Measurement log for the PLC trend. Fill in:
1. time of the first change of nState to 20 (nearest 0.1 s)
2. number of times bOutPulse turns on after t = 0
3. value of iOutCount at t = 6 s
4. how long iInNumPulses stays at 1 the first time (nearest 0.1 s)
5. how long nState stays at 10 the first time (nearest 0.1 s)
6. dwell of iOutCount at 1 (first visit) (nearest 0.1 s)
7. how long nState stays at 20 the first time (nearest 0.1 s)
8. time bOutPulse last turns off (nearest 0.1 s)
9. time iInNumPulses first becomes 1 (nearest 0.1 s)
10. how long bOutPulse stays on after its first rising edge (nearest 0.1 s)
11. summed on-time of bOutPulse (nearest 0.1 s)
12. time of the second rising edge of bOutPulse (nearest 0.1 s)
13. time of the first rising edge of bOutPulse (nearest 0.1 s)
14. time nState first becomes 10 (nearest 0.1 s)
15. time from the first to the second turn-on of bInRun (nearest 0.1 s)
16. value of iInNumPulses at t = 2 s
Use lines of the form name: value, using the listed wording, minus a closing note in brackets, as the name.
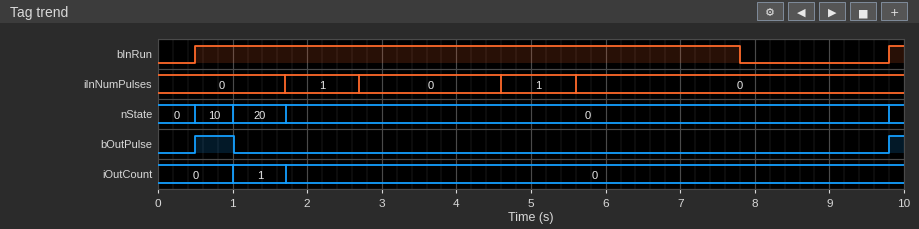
time of the first change of nState to 20: 1.0 s
number of times bOutPulse turns on after t = 0: 2
value of iOutCount at t = 6 s: 0
how long iInNumPulses stays at 1 the first time: 1.0 s
how long nState stays at 10 the first time: 0.5 s
dwell of iOutCount at 1 (first visit): 0.7 s
how long nState stays at 20 the first time: 0.7 s
time bOutPulse last turns off: 1.0 s
time iInNumPulses first becomes 1: 1.7 s
how long bOutPulse stays on after its first rising edge: 0.5 s
summed on-time of bOutPulse: 0.7 s
time of the second rising edge of bOutPulse: 9.8 s
time of the first rising edge of bOutPulse: 0.5 s
time nState first becomes 10: 0.5 s
time from the first to the second turn-on of bInRun: 9.3 s
value of iInNumPulses at t = 2 s: 1
